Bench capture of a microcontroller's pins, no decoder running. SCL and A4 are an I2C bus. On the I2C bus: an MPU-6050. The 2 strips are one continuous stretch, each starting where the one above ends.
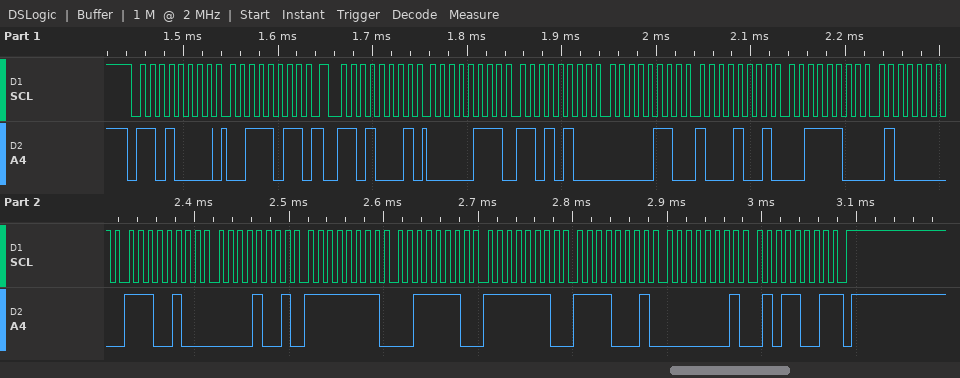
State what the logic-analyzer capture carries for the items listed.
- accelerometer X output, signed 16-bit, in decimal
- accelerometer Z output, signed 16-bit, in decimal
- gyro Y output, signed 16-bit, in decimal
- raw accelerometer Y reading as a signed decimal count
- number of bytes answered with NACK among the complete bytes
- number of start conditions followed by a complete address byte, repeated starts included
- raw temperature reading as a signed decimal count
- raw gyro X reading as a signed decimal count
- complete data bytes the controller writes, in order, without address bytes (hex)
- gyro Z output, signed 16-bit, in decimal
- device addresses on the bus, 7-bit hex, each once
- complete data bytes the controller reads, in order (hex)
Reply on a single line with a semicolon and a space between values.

2004; 15424; -271; 1673; 1; 2; -7159; -194; 3B; 345; 0x68; 07 D4 06 89 3C 40 E4 09 FF 3E FE F1 01 59
